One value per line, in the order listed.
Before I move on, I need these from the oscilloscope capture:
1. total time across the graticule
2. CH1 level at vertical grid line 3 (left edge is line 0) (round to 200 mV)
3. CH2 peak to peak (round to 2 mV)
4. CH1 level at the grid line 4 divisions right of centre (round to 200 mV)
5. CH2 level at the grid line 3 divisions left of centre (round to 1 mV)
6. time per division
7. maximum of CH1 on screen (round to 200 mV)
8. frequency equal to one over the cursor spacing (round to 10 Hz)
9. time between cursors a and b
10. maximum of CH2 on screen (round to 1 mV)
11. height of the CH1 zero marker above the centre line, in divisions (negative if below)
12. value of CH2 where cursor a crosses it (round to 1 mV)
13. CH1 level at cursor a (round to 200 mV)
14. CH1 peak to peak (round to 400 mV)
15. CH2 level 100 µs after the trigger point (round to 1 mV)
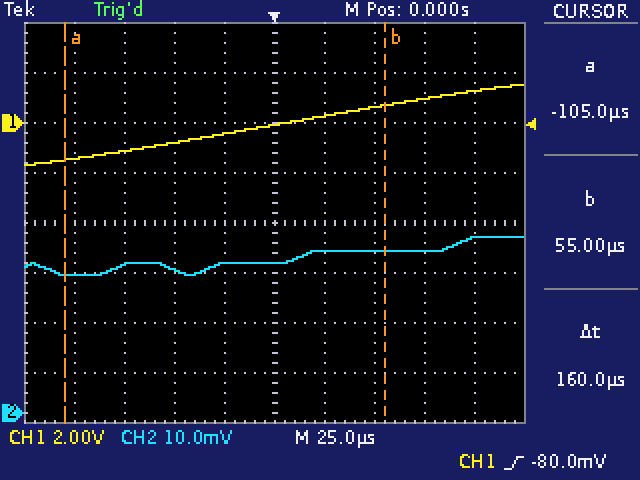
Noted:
250 µs
-800 mV
8 mV
1.2 V
30 mV
25 µs
1.6 V
6.25 kHz
160 µs
35 mV
+2.0 div
28 mV
-1.4 V
3.2 V
35 mV
